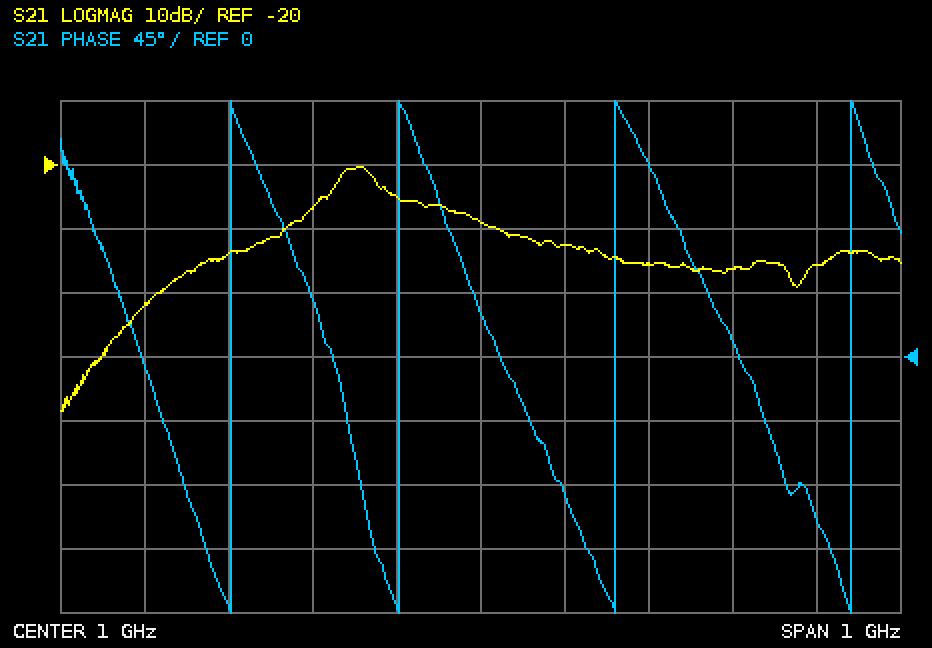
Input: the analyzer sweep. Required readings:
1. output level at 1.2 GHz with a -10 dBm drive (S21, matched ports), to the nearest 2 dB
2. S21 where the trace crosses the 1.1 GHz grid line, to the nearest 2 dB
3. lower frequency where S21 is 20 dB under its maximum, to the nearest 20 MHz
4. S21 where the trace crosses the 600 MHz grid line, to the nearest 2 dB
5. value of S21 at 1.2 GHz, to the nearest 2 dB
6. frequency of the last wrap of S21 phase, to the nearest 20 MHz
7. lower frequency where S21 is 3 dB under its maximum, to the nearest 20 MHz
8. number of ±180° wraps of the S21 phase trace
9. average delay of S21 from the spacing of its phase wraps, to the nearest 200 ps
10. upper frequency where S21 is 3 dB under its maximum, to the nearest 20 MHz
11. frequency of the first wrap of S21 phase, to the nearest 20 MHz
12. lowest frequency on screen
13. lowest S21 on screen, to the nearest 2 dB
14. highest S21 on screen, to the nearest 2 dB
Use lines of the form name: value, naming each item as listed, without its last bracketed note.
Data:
output level at 1.2 GHz with a -10 dBm drive (S21, matched ports), to the nearest 2 dB: -46 dBm
S21 where the trace crosses the 1.1 GHz grid line, to the nearest 2 dB: -32 dB
lower frequency where S21 is 20 dB under its maximum, to the nearest 20 MHz: 620 MHz
S21 where the trace crosses the 600 MHz grid line, to the nearest 2 dB: -42 dB
value of S21 at 1.2 GHz, to the nearest 2 dB: -36 dB
frequency of the last wrap of S21 phase, to the nearest 20 MHz: 1.44 GHz
lower frequency where S21 is 3 dB under its maximum, to the nearest 20 MHz: 820 MHz
number of ±180° wraps of the S21 phase trace: 4
average delay of S21 from the spacing of its phase wraps, to the nearest 200 ps: 4.0 ns
upper frequency where S21 is 3 dB under its maximum, to the nearest 20 MHz: 880 MHz
frequency of the first wrap of S21 phase, to the nearest 20 MHz: 700 MHz
lowest frequency on screen: 500 MHz
lowest S21 on screen, to the nearest 2 dB: -58 dB
highest S21 on screen, to the nearest 2 dB: -20 dB
